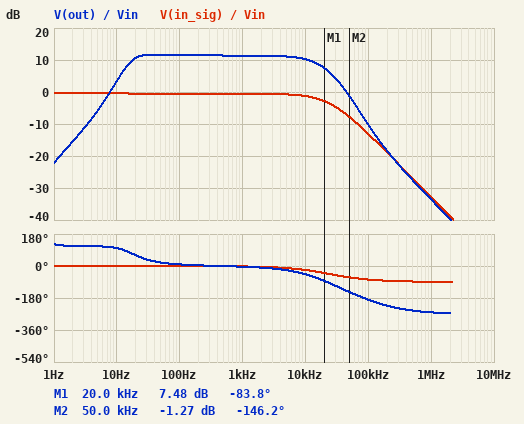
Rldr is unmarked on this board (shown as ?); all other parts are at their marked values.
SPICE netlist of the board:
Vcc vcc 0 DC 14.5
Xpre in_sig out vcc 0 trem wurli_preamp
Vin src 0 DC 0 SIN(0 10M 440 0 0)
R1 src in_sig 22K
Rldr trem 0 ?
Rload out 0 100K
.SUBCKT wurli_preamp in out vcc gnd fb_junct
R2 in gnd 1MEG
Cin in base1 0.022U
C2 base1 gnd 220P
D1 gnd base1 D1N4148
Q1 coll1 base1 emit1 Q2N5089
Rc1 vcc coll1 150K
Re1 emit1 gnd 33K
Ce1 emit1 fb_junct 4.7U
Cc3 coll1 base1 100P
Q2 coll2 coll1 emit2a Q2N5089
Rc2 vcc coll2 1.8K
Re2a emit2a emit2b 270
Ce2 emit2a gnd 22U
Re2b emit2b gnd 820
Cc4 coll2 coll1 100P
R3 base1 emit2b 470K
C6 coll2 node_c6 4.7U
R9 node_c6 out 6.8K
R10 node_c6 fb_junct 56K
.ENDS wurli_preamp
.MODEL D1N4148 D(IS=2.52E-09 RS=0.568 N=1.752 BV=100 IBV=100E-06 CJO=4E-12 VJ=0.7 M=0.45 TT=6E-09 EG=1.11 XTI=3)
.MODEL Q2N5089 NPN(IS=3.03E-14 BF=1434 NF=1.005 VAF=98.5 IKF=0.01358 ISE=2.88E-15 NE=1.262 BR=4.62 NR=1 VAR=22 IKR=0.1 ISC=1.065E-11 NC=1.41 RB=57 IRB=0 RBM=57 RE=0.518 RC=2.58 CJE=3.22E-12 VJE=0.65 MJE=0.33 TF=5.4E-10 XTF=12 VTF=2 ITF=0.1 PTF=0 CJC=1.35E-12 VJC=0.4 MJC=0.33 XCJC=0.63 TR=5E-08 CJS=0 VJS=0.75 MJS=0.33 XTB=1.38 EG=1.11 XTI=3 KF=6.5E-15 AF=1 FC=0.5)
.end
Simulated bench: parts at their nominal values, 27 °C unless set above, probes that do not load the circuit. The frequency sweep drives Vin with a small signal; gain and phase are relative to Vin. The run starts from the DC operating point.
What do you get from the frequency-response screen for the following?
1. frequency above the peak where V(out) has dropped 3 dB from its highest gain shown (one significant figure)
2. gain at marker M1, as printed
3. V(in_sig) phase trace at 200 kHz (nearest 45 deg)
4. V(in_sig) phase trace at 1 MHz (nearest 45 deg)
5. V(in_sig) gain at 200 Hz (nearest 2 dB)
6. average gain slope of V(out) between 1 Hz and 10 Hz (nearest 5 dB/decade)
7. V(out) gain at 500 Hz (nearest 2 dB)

20 kHz
7.48 dB
-90 deg
-90 deg
0 dB
25 dB/decade
12 dB
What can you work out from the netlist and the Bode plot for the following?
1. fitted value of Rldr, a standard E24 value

30 kΩ
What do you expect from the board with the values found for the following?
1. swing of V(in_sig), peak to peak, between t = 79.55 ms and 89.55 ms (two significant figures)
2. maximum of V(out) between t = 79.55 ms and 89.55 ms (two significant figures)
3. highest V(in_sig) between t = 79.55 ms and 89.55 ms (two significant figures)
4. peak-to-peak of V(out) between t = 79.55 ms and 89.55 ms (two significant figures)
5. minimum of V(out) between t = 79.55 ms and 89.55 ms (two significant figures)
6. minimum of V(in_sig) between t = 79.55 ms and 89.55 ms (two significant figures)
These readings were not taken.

19 mV
37 mV
9.4 mV
74 mV
-37 mV
-9.4 mV
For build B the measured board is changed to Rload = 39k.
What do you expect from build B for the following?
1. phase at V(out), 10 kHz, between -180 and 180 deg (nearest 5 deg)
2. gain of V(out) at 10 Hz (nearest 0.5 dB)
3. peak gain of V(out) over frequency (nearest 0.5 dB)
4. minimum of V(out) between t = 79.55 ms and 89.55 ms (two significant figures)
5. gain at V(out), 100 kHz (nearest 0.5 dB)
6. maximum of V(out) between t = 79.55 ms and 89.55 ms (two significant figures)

-45 deg
2.5 dB
11.0 dB
-34 mV
-11.0 dB
34 mV
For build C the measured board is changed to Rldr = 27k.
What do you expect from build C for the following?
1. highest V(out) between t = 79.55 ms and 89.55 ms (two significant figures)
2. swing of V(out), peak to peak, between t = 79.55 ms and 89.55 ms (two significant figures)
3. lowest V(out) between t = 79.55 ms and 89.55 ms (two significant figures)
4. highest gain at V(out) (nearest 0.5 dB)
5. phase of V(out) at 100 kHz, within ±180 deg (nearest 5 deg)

39 mV
78 mV
-39 mV
12.0 dB
170 deg
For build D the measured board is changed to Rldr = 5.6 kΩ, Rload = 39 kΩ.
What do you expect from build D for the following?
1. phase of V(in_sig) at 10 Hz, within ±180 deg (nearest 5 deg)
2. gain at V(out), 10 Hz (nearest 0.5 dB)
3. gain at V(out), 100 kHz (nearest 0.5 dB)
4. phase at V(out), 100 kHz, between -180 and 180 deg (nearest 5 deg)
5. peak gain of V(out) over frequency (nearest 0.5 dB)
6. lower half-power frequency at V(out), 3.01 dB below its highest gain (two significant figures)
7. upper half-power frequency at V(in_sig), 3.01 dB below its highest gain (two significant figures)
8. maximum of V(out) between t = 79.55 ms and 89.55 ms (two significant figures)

0 deg
5.5 dB
-4.5 dB
-170 deg
21.5 dB
21 Hz
21 kHz
94 mV
